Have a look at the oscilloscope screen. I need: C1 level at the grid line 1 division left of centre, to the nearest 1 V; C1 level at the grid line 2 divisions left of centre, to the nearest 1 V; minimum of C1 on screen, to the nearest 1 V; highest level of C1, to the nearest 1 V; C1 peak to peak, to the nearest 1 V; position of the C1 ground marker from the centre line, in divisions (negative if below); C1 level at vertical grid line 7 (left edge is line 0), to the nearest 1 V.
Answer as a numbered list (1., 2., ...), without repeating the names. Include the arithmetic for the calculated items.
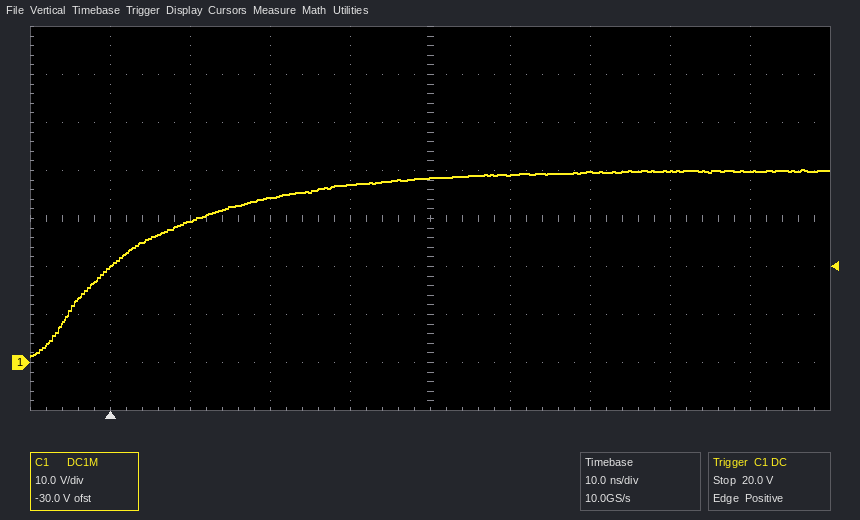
1. 37 V
2. 34 V
3. 1 V
4. 40 V
5. 40 V − (1 V) = 39 V
6. -3.0 div
7. 40 V
